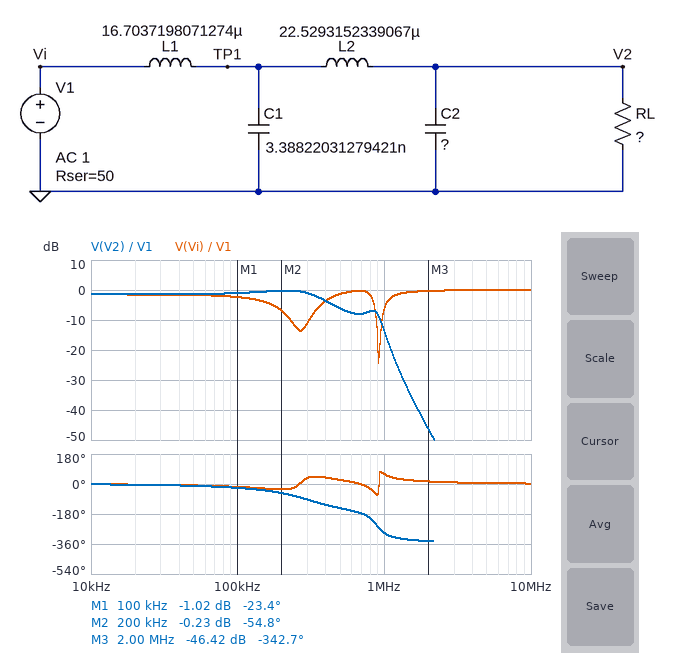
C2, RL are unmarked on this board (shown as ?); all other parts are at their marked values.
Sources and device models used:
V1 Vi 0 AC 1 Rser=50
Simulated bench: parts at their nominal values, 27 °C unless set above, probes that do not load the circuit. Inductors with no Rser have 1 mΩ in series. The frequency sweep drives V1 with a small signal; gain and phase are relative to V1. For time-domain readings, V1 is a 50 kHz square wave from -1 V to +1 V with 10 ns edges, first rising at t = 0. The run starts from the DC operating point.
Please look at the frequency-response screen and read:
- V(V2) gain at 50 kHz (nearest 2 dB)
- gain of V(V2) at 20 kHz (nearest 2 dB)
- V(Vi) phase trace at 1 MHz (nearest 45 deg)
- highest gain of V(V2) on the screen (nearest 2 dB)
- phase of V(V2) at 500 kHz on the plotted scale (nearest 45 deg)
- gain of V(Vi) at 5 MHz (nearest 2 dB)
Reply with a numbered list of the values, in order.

1. -2 dB
2. -2 dB
3. 45 deg
4. 0 dB
5. -135 deg
6. 0 dB
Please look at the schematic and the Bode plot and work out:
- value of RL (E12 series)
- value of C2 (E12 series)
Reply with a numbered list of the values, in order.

1. 270 Ω
2. 8.2 nF
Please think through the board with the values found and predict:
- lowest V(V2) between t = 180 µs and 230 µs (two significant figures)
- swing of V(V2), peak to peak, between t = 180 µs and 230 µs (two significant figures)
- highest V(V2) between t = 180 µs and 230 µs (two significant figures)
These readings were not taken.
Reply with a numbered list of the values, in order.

1. -1.1 V
2. 2.2 V
3. 1.1 V
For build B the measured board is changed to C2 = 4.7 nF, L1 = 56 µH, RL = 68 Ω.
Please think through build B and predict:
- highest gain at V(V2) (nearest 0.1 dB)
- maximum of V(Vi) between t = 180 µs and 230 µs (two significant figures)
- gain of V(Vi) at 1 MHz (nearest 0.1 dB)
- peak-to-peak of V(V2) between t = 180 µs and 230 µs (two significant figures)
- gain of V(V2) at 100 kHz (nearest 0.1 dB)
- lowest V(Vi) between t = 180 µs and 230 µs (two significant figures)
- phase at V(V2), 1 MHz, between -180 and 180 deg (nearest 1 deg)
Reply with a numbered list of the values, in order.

1. -4.8 dB
2. 1.4 V
3. -0.2 dB
4. 1.3 V
5. -5.0 dB
6. -1.4 V
7. 49 deg
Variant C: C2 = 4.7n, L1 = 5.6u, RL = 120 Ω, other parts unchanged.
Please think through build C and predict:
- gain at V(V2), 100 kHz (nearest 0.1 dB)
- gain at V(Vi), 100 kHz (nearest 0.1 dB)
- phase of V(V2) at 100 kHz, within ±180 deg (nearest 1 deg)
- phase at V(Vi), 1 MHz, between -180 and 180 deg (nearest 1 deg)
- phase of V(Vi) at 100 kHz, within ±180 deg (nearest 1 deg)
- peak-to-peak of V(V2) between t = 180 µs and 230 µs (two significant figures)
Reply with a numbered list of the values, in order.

1. -2.9 dB
2. -3.4 dB
3. -16 deg
4. -44 deg
5. -8 deg
6. 1.8 V
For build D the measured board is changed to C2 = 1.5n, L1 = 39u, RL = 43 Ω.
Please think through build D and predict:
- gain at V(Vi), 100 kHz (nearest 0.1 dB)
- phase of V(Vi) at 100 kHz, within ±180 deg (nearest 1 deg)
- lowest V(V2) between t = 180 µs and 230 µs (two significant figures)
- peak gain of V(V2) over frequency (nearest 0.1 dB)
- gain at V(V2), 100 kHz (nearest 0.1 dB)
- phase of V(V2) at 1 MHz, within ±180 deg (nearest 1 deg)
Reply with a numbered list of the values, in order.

1. -5.1 dB
2. 17 deg
3. -480 mV
4. -6.7 dB
5. -7.2 dB
6. 112 deg
